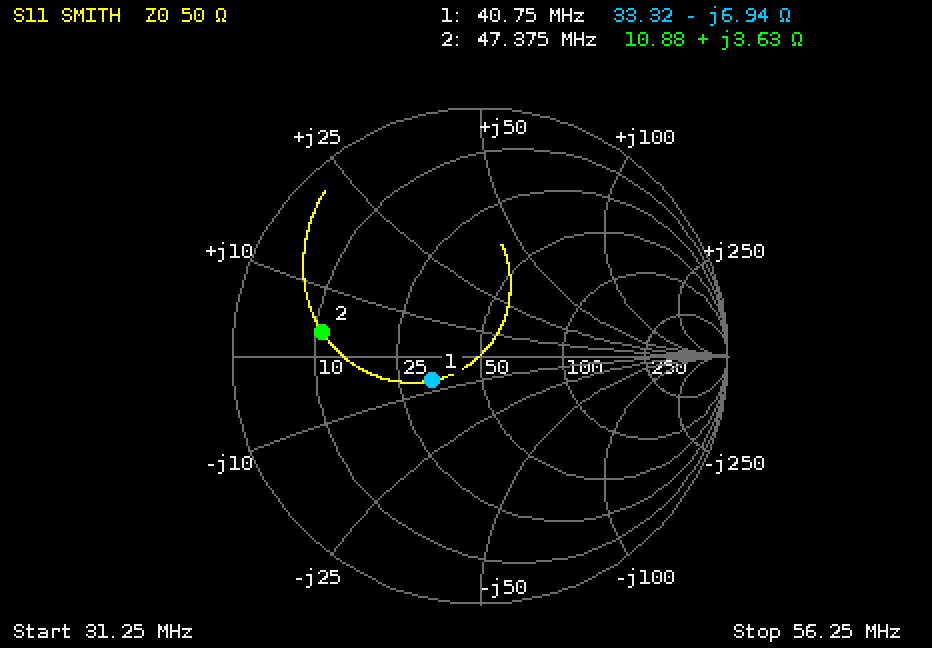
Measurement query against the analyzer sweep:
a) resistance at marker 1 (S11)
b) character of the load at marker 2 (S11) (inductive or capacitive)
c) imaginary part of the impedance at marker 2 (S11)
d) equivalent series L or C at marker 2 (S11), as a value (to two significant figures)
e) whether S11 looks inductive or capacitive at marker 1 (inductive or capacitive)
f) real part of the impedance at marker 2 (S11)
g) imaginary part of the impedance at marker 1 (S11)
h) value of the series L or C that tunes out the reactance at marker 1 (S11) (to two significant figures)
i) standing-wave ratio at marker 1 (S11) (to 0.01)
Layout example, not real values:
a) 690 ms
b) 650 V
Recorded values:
a) 33.32 Ω
b) inductive
c) +3.63 Ω
d) 12 nH
e) capacitive
f) 10.88 Ω
g) -6.94 Ω
h) 27 nH
i) 1.55
